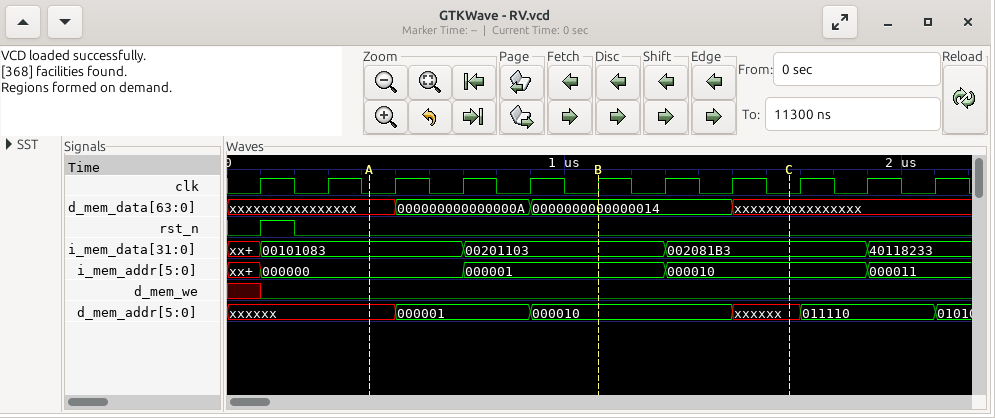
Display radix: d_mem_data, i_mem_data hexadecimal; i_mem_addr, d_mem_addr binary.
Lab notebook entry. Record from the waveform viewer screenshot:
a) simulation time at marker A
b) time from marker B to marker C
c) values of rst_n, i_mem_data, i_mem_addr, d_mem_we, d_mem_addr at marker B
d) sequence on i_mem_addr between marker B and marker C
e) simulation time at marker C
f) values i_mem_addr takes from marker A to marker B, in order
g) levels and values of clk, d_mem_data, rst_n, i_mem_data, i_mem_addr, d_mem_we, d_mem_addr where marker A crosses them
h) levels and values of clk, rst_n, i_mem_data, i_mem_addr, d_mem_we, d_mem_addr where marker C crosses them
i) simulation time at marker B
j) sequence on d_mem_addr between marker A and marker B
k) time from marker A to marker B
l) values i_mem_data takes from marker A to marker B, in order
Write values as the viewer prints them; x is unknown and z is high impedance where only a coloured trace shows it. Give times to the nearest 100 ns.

400 ns
600 ns
rst_n=0, i_mem_data=00201103, i_mem_addr=000001, d_mem_we=0, d_mem_addr=000010
000001, 000010
1700 ns
000000, 000001
clk=0, d_mem_data=xxxxxxxxxxxxxxxx, rst_n=0, i_mem_data=00101083, i_mem_addr=000000, d_mem_we=0, d_mem_addr=xxxxxx
clk=0, rst_n=0, i_mem_data=002081B3, i_mem_addr=000010, d_mem_we=0, d_mem_addr=xxxxxx
1100 ns
xxxxxx, 000001, 000010
700 ns
00101083, 00201103
